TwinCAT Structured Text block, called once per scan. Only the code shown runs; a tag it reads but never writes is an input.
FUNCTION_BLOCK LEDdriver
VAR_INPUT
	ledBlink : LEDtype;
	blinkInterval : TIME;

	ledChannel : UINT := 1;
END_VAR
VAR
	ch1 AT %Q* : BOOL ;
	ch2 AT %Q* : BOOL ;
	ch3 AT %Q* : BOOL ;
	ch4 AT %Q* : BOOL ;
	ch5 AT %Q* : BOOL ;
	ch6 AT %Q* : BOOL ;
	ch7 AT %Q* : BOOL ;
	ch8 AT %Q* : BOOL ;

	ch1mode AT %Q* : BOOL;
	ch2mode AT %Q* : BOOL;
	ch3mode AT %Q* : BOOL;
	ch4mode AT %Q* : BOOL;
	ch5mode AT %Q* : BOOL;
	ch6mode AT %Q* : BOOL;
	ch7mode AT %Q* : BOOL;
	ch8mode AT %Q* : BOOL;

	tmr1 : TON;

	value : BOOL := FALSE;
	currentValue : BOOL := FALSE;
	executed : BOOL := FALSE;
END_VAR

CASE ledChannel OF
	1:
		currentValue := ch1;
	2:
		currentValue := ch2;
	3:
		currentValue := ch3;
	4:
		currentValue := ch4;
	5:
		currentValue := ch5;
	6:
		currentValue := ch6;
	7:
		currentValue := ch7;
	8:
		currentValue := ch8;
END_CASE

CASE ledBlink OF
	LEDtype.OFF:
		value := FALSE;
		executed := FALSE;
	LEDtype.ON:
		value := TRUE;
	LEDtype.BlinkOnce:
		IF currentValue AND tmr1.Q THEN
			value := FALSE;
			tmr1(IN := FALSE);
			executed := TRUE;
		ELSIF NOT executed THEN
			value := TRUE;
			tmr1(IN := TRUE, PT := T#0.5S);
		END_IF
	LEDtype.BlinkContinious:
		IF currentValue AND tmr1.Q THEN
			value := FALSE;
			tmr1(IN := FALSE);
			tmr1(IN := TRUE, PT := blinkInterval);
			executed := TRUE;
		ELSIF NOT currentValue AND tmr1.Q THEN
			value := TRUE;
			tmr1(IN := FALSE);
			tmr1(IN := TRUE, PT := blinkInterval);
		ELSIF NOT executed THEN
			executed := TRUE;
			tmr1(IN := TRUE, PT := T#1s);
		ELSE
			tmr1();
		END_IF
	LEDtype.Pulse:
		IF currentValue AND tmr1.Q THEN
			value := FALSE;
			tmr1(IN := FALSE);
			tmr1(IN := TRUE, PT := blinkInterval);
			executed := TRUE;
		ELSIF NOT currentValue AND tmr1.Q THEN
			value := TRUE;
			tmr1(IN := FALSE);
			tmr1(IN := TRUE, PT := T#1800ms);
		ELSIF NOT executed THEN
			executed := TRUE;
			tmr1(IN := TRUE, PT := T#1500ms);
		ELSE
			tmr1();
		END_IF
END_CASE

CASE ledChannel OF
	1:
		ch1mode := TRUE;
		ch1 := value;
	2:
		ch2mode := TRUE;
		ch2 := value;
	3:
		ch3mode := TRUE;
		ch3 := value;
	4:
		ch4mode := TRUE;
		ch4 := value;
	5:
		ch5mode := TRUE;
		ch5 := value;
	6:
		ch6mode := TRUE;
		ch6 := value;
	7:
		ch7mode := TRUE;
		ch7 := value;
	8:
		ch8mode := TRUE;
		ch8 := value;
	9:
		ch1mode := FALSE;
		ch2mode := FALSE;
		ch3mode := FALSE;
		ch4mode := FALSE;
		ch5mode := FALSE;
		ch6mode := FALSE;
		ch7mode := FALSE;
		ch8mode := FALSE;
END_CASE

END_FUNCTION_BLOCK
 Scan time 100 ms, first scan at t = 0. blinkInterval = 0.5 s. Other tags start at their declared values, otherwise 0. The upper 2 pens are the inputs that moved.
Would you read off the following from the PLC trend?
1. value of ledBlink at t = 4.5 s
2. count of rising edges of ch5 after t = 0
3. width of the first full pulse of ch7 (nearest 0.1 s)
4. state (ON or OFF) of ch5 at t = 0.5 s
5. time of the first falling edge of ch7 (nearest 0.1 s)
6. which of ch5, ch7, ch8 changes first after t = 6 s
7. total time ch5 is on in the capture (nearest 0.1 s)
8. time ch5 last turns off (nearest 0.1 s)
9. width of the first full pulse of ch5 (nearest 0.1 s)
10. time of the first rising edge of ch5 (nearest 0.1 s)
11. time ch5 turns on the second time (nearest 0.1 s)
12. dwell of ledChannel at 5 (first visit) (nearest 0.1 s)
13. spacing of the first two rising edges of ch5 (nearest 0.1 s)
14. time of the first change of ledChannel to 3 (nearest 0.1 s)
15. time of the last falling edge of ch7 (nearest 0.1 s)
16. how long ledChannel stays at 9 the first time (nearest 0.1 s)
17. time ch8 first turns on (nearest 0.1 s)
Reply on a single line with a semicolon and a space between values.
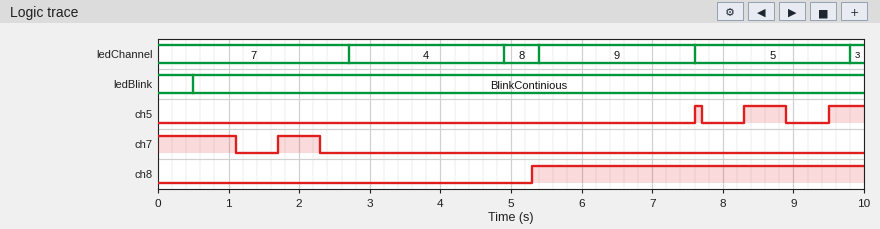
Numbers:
BlinkContinious; 3; 0.6 s; OFF; 1.1 s; ch5; 1.2 s; 8.9 s; 0.1 s; 7.6 s; 8.3 s; 2.2 s; 0.7 s; 9.8 s; 2.3 s; 2.2 s; 5.3 s
